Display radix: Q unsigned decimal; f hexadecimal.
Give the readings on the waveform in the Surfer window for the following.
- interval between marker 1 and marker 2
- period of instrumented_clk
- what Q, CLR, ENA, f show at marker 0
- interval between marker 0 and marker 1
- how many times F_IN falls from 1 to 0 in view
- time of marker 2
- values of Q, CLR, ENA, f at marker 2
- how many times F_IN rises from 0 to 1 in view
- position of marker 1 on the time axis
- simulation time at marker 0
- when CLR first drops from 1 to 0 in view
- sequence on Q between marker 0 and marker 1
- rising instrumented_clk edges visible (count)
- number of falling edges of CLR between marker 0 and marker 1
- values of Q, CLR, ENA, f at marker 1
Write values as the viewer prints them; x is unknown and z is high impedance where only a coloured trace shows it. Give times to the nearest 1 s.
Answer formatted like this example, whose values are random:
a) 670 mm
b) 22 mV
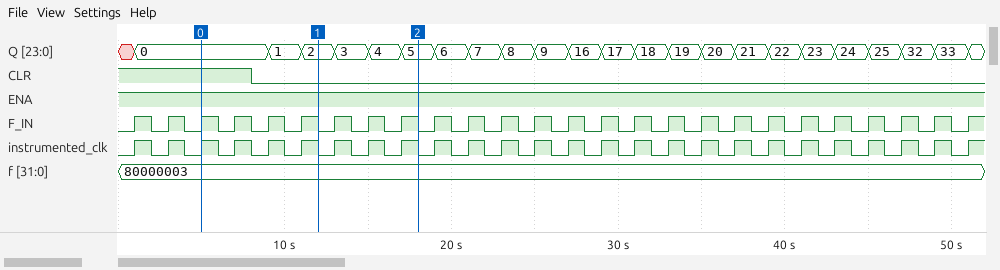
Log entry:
a) 6 s
b) 2 s
c) Q=0, CLR=1, ENA=1, f=80000003
d) 7 s
e) 25
f) 18 s
g) Q=5, CLR=0, ENA=1, f=80000003
h) 26
i) 12 s
j) 5 s
k) 8 s
l) 0, 1, 2
m) 26
n) 1
o) Q=2, CLR=0, ENA=1, f=80000003
